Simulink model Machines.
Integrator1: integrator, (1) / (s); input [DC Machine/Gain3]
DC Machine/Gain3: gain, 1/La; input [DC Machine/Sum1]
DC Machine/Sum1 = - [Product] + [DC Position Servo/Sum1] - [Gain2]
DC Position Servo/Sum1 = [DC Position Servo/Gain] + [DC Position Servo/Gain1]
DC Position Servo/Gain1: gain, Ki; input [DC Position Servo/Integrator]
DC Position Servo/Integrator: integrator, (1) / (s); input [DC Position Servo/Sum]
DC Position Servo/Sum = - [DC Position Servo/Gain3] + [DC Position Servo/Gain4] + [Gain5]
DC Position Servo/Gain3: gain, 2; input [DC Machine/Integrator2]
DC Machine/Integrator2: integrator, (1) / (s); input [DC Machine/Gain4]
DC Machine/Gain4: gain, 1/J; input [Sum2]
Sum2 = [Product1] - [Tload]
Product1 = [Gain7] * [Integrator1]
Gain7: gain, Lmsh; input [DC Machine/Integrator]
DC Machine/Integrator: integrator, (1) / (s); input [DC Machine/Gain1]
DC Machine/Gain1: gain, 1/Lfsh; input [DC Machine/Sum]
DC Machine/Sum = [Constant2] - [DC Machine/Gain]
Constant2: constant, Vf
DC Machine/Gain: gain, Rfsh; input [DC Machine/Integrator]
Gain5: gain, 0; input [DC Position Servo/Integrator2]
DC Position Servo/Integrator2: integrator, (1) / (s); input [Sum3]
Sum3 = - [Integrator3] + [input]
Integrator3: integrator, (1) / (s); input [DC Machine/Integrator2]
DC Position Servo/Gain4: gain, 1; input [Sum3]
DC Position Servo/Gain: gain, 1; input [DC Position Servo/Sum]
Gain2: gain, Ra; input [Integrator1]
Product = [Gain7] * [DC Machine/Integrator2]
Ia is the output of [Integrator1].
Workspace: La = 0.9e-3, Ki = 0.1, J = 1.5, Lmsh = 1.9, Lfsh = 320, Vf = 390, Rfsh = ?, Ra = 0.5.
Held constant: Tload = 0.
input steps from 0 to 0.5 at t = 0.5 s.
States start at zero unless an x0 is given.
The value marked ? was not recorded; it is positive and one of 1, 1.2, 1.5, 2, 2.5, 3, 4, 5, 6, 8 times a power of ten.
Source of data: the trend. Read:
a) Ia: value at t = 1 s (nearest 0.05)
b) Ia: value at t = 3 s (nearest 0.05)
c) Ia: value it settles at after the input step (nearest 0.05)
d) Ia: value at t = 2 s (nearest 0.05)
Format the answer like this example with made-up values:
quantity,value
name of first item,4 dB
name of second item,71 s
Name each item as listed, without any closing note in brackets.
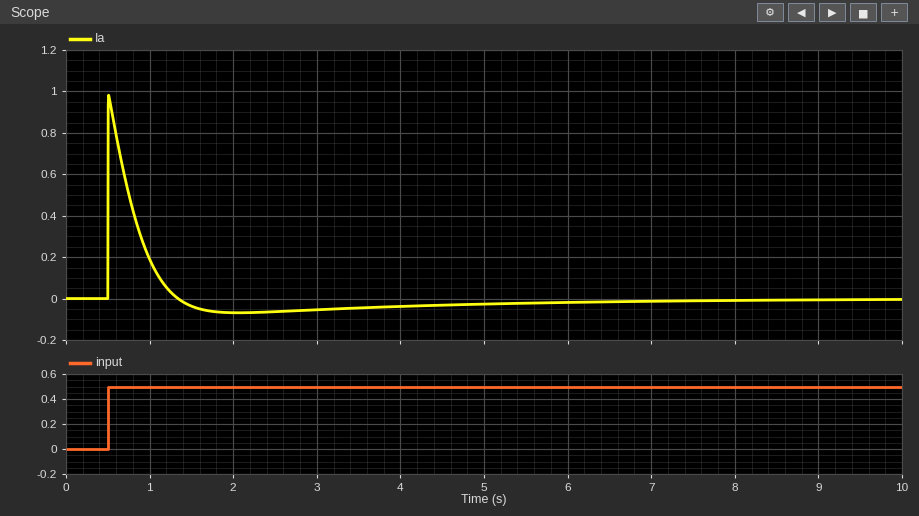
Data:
quantity,value
Ia: value at t = 1 s,0.20
Ia: value at t = 3 s,-0.05
Ia: value it settles at after the input step,0.00
Ia: value at t = 2 s,-0.05
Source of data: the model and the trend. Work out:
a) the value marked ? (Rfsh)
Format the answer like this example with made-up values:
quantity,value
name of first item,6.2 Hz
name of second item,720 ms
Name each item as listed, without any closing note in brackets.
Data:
quantity,value
the value marked ?,800
